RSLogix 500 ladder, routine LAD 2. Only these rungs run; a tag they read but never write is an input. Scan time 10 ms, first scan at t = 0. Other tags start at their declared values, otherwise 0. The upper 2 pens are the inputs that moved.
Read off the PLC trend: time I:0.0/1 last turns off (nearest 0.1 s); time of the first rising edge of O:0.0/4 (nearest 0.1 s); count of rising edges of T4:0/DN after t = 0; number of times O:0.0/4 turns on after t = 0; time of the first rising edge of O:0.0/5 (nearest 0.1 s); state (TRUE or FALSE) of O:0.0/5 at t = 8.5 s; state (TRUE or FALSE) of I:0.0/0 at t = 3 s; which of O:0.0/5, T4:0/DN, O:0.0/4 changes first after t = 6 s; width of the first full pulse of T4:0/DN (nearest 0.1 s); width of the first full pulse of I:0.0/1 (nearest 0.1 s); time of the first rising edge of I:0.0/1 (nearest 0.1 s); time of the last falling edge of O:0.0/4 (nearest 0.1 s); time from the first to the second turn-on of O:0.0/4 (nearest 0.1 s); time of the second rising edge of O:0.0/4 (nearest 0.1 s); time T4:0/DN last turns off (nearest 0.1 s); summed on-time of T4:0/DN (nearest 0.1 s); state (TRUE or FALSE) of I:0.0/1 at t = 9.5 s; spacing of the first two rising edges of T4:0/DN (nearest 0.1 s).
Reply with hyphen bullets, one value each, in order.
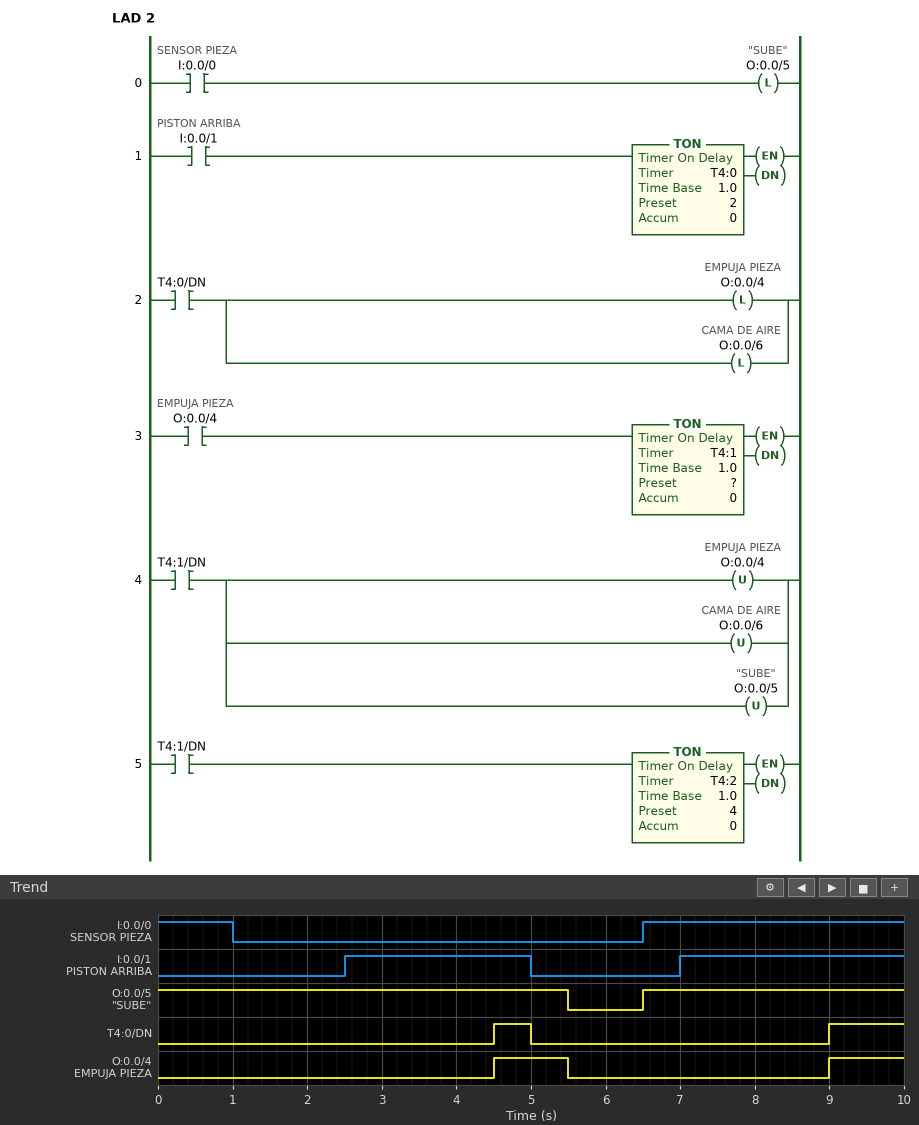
- 5.0 s
- 4.5 s
- 2
- 2
- 6.5 s
- TRUE
- FALSE
- O:0.0/5
- 0.5 s
- 2.5 s
- 2.5 s
- 5.5 s
- 4.5 s
- 9.0 s
- 5.0 s
- 1.5 s
- TRUE
- 4.5 s
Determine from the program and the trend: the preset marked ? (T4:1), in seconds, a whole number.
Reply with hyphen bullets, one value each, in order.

- 1 s
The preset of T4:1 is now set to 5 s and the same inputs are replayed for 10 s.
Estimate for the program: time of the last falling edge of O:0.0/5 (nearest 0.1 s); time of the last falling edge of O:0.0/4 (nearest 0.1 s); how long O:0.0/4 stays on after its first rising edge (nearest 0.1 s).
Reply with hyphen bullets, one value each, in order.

- 9.5 s
- 9.5 s
- 5.0 s
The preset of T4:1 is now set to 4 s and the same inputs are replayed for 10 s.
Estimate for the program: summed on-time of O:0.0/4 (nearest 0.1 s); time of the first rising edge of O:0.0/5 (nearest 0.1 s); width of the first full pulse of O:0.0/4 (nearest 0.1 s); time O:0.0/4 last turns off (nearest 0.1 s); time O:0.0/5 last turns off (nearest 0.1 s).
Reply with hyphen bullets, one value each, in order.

- 5.0 s
- 8.5 s
- 4.0 s
- 8.5 s
- 8.5 s
